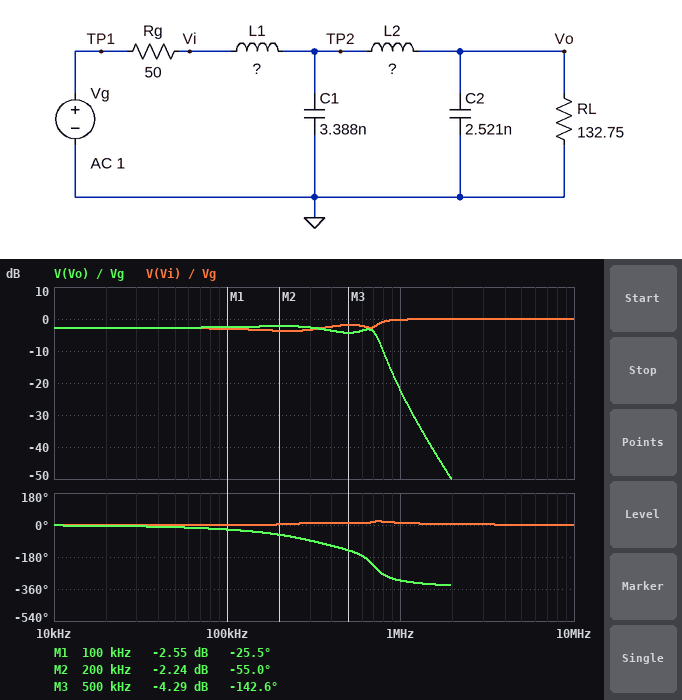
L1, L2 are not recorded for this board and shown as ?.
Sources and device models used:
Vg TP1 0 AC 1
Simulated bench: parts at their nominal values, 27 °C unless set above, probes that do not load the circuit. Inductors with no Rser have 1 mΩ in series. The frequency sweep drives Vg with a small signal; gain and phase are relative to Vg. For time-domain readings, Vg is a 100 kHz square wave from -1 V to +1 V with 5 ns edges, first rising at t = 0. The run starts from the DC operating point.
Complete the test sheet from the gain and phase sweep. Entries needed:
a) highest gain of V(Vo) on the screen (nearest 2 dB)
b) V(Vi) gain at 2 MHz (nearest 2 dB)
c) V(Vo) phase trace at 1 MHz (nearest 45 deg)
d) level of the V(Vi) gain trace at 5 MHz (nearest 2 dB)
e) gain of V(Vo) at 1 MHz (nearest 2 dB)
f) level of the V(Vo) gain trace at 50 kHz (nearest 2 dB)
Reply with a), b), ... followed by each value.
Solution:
a) -2 dB
b) 0 dB
c) -315 deg
d) 0 dB
e) -22 dB
f) -2 dB
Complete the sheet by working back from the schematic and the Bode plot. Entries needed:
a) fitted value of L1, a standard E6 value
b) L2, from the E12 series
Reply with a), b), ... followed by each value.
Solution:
a) 47 µH
b) 39 µH
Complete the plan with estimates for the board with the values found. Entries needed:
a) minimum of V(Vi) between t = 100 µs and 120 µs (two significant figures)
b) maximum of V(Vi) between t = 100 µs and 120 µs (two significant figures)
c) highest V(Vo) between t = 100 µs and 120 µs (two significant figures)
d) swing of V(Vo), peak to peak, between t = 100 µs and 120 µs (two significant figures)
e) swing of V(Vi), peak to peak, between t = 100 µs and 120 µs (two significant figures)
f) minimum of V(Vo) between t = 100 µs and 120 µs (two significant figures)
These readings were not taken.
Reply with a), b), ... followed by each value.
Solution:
a) -1.3 V
b) 1.3 V
c) 940 mV
d) 1.9 V
e) 2.5 V
f) -940 mV
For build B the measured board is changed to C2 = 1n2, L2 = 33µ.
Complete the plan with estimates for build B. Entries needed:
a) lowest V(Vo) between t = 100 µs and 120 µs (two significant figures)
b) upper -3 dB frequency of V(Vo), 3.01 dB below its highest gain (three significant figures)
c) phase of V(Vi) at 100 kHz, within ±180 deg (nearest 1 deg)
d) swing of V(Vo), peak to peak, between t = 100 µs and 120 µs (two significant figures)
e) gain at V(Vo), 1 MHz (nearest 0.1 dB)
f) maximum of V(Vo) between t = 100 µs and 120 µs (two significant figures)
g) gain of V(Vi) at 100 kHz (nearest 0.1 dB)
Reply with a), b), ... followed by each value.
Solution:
a) -900 mV
b) 655 kHz
c) 0 deg
d) 1.8 V
e) -16.0 dB
f) 900 mV
g) -2.9 dB
